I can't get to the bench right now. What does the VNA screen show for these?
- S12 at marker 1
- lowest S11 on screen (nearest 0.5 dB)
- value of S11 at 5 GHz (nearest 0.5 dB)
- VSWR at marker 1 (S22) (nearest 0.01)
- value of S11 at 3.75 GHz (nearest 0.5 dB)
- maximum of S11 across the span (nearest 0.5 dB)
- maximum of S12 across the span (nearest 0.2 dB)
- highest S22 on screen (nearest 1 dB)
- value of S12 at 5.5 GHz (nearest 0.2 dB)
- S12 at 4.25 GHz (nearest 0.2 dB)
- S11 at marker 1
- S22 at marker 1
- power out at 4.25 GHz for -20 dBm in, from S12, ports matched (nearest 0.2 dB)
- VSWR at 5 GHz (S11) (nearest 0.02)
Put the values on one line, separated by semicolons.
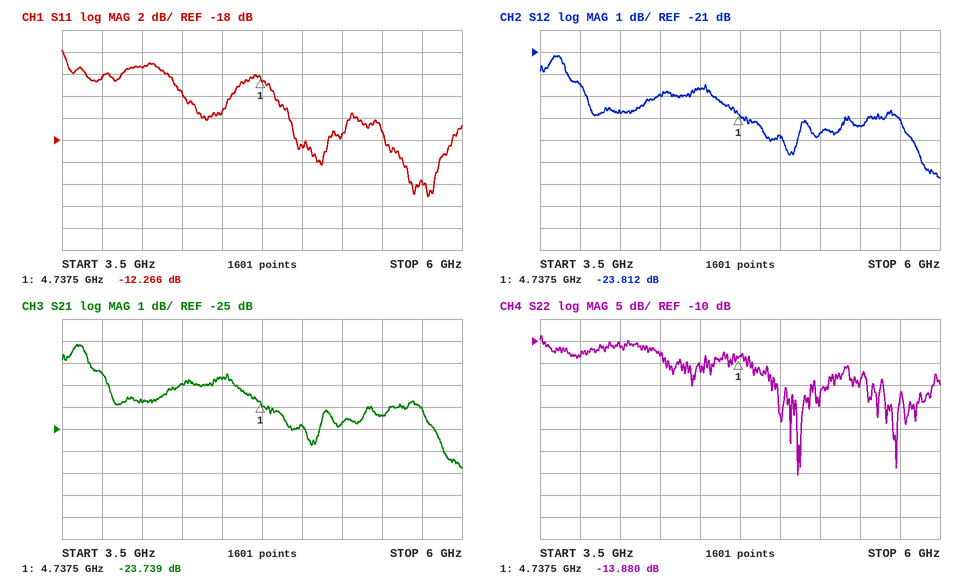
-23.812 dB; -23.0 dB; -18.5 dB; 1.51; -12.5 dB; -10.0 dB; -21.2 dB; -9 dB; -24.4 dB; -23.0 dB; -12.266 dB; -13.880 dB; -43.0 dBm; 1.26
